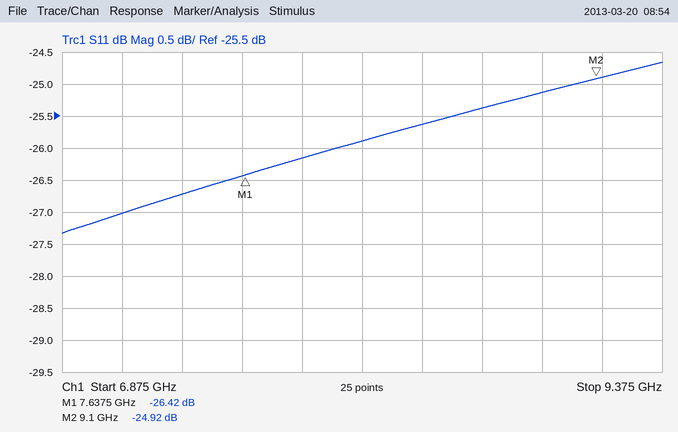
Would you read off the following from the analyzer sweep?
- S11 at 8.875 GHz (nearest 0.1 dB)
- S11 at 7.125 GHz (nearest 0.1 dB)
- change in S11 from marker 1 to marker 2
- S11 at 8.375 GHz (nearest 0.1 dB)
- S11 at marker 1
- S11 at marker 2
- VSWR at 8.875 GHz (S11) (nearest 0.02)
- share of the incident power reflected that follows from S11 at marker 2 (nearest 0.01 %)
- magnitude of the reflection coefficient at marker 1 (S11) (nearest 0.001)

-25.1 dB
-27.0 dB
1.50 dB
-25.6 dB
-26.42 dB
-24.92 dB
1.12
0.32 %
0.048
